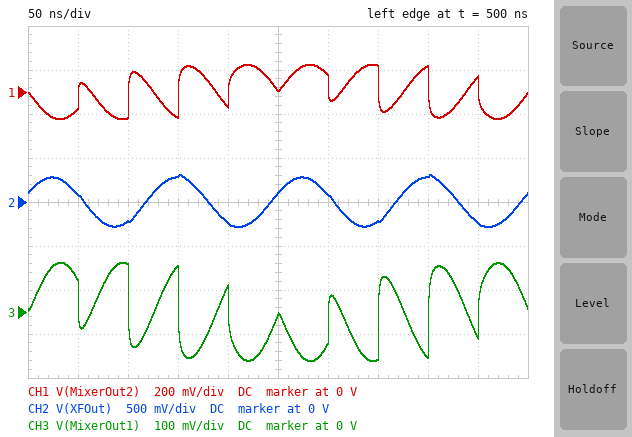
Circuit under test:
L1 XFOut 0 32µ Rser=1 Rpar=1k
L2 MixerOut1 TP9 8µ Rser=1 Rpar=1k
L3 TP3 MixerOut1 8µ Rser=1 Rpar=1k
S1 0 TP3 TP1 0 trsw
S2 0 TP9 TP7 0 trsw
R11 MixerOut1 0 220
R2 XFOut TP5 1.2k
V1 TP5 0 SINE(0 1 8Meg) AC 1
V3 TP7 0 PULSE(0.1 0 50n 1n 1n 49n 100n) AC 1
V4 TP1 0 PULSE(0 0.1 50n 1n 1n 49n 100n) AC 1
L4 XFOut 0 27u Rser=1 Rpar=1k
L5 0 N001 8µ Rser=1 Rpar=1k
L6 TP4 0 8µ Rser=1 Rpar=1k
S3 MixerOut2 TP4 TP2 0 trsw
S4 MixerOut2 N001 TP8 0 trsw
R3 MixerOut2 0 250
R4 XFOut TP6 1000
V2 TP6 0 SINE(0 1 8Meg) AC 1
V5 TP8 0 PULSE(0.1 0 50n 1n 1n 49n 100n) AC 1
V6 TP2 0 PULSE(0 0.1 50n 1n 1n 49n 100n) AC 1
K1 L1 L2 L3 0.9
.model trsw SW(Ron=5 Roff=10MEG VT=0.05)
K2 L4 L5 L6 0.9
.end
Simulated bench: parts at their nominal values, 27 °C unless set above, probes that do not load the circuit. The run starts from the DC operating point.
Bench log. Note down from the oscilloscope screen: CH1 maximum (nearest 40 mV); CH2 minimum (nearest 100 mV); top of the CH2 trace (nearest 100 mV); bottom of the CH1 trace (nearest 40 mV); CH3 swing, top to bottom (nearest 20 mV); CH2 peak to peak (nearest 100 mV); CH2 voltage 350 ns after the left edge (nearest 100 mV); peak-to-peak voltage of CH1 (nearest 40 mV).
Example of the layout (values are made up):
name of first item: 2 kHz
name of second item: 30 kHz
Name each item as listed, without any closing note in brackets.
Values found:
CH1 maximum: 120 mV
CH2 minimum: -300 mV
top of the CH2 trace: 300 mV
bottom of the CH1 trace: -120 mV
CH3 swing, top to bottom: 220 mV
CH2 peak to peak: 600 mV
CH2 voltage 350 ns after the left edge: -200 mV
peak-to-peak voltage of CH1: 240 mV
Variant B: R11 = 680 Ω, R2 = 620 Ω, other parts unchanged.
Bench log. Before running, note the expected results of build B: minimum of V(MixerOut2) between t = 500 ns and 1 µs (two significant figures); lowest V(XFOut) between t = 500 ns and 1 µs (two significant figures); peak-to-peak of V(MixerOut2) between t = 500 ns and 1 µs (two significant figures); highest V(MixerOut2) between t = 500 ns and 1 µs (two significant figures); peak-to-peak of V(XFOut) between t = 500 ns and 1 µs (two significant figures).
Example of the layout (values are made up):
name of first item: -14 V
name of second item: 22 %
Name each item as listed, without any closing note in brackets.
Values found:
minimum of V(MixerOut2) between t = 500 ns and 1 µs: -170 mV
lowest V(XFOut) between t = 500 ns and 1 µs: -390 mV
peak-to-peak of V(MixerOut2) between t = 500 ns and 1 µs: 340 mV
highest V(MixerOut2) between t = 500 ns and 1 µs: 170 mV
peak-to-peak of V(XFOut) between t = 500 ns and 1 µs: 790 mV
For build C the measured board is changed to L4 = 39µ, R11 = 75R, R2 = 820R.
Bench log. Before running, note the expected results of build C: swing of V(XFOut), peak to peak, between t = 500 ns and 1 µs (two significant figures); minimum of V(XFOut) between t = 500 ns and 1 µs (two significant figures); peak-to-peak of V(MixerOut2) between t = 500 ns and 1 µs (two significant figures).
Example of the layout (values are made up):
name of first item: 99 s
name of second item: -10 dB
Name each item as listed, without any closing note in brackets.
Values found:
swing of V(XFOut), peak to peak, between t = 500 ns and 1 µs: 670 mV
minimum of V(XFOut) between t = 500 ns and 1 µs: -320 mV
peak-to-peak of V(MixerOut2) between t = 500 ns and 1 µs: 230 mV
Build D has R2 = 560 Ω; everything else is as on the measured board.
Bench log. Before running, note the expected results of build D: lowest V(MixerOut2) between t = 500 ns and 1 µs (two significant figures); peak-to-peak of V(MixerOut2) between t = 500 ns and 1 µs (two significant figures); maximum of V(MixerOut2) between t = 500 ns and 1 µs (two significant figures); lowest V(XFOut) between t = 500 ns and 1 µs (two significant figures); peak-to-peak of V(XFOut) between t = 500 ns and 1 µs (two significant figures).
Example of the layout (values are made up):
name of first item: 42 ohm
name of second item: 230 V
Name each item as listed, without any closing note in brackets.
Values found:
lowest V(MixerOut2) between t = 500 ns and 1 µs: -170 mV
peak-to-peak of V(MixerOut2) between t = 500 ns and 1 µs: 330 mV
maximum of V(MixerOut2) between t = 500 ns and 1 µs: 170 mV
lowest V(XFOut) between t = 500 ns and 1 µs: -380 mV
peak-to-peak of V(XFOut) between t = 500 ns and 1 µs: 780 mV
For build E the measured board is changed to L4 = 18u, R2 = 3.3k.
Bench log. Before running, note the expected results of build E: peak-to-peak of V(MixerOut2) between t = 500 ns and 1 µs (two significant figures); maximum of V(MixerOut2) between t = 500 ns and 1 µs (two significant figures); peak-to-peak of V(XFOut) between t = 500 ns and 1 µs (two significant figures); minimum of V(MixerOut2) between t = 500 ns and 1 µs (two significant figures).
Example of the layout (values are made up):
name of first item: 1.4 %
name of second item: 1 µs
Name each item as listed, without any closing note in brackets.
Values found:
peak-to-peak of V(MixerOut2) between t = 500 ns and 1 µs: 210 mV
maximum of V(MixerOut2) between t = 500 ns and 1 µs: 100 mV
peak-to-peak of V(XFOut) between t = 500 ns and 1 µs: 410 mV
minimum of V(MixerOut2) between t = 500 ns and 1 µs: -100 mV
